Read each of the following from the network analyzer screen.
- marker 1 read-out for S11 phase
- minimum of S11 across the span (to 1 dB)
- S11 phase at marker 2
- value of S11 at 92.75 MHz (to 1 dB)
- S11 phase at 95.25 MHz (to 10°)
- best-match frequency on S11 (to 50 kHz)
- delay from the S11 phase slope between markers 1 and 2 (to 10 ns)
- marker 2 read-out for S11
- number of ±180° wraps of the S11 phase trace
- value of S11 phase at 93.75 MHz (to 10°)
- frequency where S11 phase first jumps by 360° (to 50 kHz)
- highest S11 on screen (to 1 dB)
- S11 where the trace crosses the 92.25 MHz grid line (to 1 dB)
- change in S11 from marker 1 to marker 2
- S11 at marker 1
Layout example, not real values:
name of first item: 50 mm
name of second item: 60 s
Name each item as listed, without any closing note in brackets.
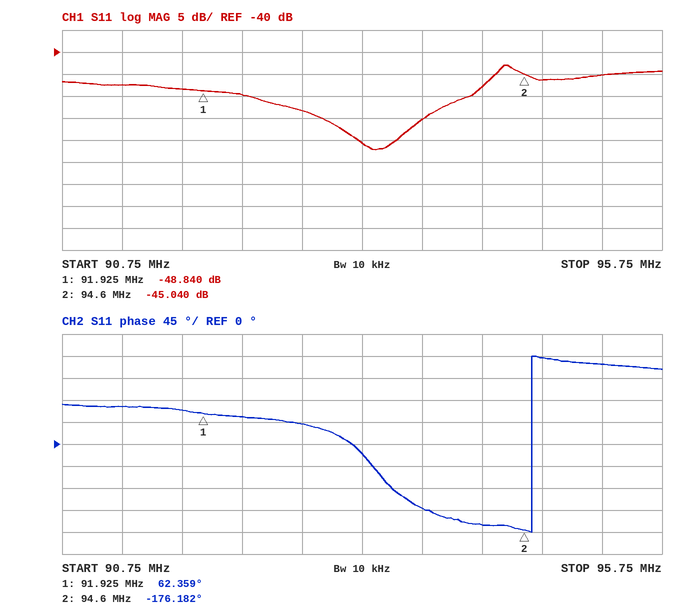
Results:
marker 1 read-out for S11 phase: 62.359°
minimum of S11 across the span: -62 dB
S11 phase at marker 2: -176.182°
value of S11 at 92.75 MHz: -53 dB
S11 phase at 95.25 MHz: 160°
best-match frequency on S11: 93.35 MHz
delay from the S11 phase slope between markers 1 and 2: 250 ns
marker 2 read-out for S11: -45.040 dB
number of ±180° wraps of the S11 phase trace: 1
value of S11 phase at 93.75 MHz: -130°
frequency where S11 phase first jumps by 360°: 94.65 MHz
highest S11 on screen: -43 dB
S11 where the trace crosses the 92.25 MHz grid line: -50 dB
change in S11 from marker 1 to marker 2: 3.800 dB
S11 at marker 1: -48.840 dB
